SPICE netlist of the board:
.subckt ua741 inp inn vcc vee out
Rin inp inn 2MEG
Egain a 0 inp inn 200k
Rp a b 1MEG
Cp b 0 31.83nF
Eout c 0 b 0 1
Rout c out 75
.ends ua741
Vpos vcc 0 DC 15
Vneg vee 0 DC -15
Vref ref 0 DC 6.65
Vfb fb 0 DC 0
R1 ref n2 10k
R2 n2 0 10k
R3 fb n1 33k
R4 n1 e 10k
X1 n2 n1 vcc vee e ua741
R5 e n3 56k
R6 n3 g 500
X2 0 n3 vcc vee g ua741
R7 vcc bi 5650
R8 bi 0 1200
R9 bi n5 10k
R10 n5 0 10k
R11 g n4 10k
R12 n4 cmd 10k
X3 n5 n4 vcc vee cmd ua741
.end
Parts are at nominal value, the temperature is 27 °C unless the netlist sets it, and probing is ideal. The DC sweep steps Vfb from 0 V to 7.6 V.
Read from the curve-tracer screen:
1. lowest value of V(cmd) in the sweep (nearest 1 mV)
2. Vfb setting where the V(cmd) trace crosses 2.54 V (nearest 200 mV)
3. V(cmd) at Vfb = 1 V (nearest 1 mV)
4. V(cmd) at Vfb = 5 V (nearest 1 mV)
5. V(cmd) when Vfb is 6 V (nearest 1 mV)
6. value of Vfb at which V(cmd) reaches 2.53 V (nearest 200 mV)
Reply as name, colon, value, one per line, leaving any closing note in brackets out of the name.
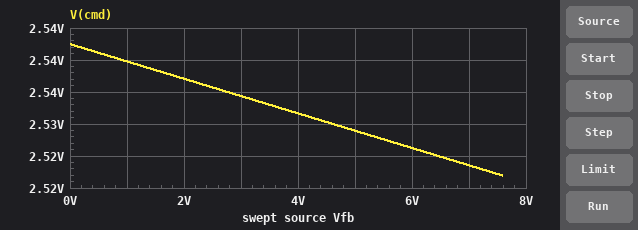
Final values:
lowest value of V(cmd) in the sweep: 2.522 V
Vfb setting where the V(cmd) trace crosses 2.54 V: 2.8 V
V(cmd) at Vfb = 1 V: 2.540 V
V(cmd) at Vfb = 5 V: 2.529 V
V(cmd) when Vfb is 6 V: 2.526 V
value of Vfb at which V(cmd) reaches 2.53 V: 4.6 V
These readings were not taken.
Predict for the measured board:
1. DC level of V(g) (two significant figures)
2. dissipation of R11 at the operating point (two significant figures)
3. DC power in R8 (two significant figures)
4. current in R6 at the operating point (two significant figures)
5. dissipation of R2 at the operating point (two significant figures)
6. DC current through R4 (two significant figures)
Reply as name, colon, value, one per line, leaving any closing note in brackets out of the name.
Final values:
DC level of V(g): -39 mV
dissipation of R11 at the operating point: 170 µW
DC power in R8: 5.2 mW
current in R6 at the operating point: 77 µA
dissipation of R2 at the operating point: 1.1 mW
DC current through R4: 100 µA
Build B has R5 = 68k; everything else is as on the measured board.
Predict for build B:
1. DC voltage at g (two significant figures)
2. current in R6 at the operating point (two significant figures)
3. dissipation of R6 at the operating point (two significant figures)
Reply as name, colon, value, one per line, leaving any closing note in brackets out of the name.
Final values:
DC voltage at g: -32 mV
current in R6 at the operating point: 64 µA
dissipation of R6 at the operating point: 2.0 µW
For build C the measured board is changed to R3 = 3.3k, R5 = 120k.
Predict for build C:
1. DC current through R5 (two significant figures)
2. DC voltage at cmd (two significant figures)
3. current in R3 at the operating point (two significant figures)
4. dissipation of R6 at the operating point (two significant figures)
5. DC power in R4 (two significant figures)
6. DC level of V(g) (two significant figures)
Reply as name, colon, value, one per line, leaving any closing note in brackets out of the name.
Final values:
DC current through R5: 110 µA
DC voltage at cmd: 2.6 V
current in R3 at the operating point: 1.0 mA
dissipation of R6 at the operating point: 6.2 µW
DC power in R4: 10 mW
DC level of V(g): -56 mV
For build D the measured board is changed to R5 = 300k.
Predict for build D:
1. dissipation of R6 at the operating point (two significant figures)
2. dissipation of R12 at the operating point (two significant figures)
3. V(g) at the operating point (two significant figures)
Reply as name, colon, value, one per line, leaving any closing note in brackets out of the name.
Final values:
dissipation of R6 at the operating point: 100 nW
dissipation of R12 at the operating point: 160 µW
V(g) at the operating point: -7.2 mV
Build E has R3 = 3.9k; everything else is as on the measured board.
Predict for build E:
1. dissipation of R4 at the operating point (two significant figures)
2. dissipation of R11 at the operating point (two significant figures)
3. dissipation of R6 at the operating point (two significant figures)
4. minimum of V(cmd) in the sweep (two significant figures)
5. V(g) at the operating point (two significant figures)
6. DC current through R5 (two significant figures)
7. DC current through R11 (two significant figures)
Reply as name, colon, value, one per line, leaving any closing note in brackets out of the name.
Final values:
dissipation of R4 at the operating point: 7.3 mW
dissipation of R11 at the operating point: 180 µW
dissipation of R6 at the operating point: 22 µW
minimum of V(cmd) in the sweep: 2.4 V
V(g) at the operating point: -110 mV
DC current through R5: 210 µA
DC current through R11: 140 µA
